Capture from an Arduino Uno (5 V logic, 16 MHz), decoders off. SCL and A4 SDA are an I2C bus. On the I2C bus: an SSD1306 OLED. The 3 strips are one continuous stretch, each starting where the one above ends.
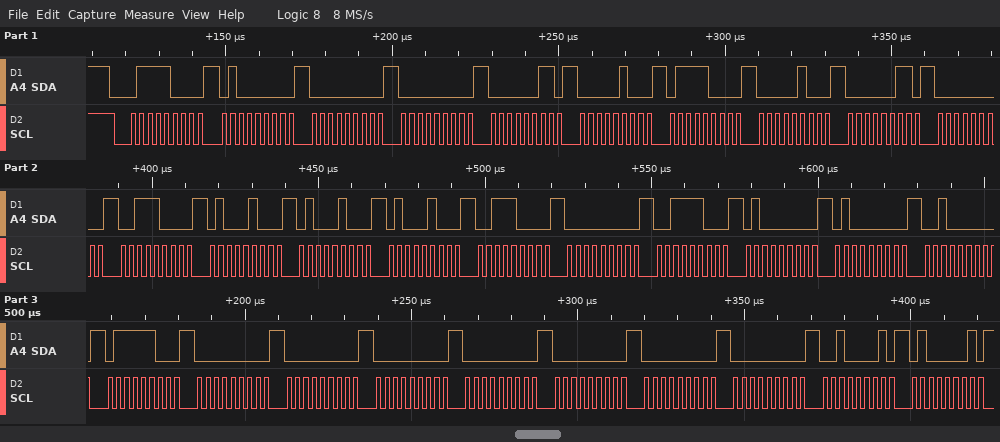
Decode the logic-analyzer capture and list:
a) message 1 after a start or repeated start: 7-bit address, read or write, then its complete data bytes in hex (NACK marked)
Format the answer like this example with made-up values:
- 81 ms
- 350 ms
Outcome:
- 0x3C write: 40 00 00 03 04 78 04 03 00 38 44 44 44 38 00 3C 40 40 20 7C 00 00 00 00 00 00 00 21 41
